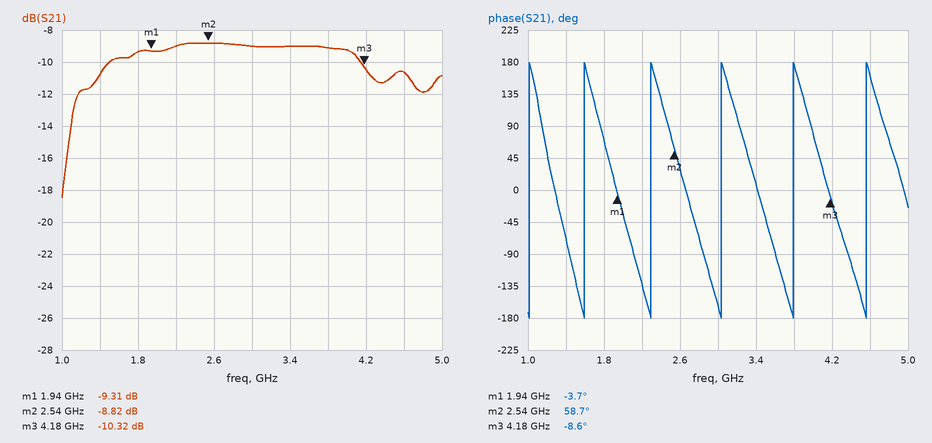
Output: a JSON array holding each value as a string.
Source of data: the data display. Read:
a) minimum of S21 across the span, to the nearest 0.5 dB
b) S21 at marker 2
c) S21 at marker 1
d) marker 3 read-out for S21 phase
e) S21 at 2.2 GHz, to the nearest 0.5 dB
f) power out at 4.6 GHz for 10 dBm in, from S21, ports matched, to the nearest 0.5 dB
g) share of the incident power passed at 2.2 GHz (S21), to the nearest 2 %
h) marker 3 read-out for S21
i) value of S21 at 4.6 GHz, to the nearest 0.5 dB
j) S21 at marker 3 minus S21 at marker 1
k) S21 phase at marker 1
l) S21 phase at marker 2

["-18.5 dB", "-8.82 dB", "-9.31 dB", "-8.6°", "-9.0 dB", "-0.5 dBm", "12 %", "-10.32 dB", "-10.5 dB", "-1.01 dB", "-3.7°", "58.7°"]
